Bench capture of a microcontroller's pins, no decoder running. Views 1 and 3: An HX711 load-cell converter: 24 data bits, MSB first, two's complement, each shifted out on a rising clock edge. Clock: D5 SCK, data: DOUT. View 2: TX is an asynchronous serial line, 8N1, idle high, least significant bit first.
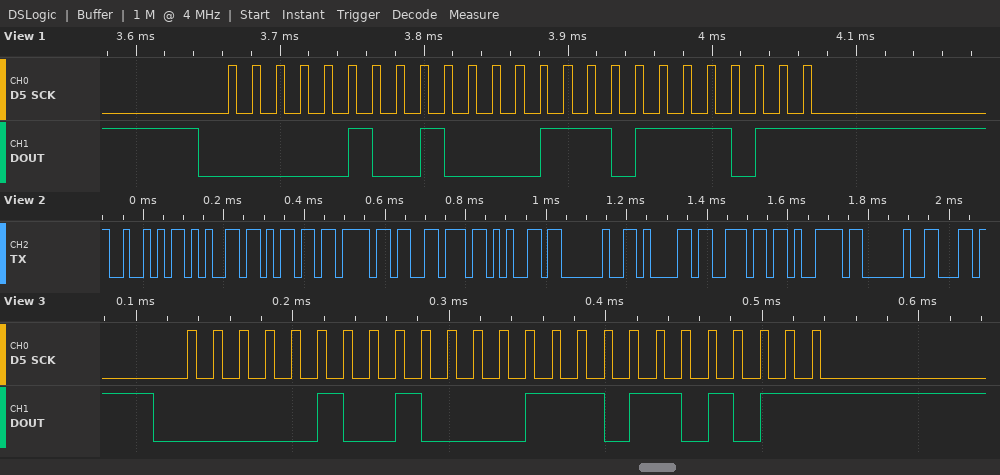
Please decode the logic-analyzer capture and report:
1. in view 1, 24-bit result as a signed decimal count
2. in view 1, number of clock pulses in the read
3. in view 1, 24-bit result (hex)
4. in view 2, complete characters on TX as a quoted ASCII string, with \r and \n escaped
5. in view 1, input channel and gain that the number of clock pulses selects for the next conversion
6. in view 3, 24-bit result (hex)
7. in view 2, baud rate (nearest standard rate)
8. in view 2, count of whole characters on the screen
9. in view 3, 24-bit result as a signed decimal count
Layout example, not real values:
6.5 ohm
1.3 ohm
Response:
296827
25
0x04877B
"Remove any "
channel A, gain 128
0x04876B
57600 baud
11
296811
